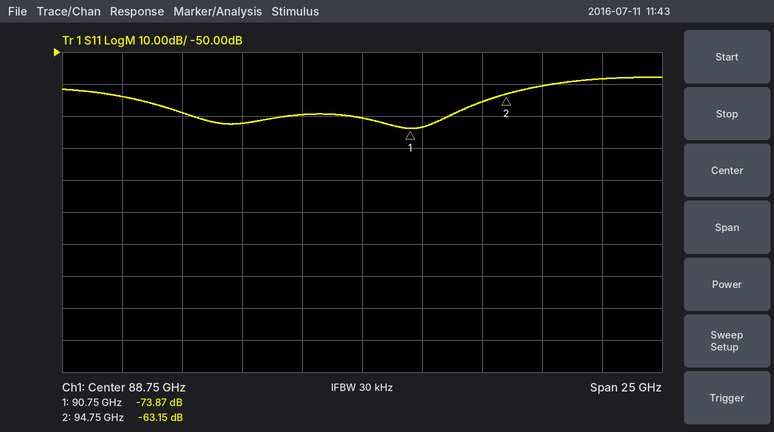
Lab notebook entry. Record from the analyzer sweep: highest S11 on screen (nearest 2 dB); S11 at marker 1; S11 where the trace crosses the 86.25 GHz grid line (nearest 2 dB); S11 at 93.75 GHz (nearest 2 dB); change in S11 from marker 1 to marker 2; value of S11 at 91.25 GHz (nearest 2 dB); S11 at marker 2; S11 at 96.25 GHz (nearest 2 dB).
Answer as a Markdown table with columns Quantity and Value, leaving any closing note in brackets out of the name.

| Quantity | Value |
|---|---|
| highest S11 on screen | -58 dB |
| S11 at marker 1 | -73.87 dB |
| S11 where the trace crosses the 86.25 GHz grid line | -70 dB |
| S11 at 93.75 GHz | -66 dB |
| change in S11 from marker 1 to marker 2 | 10.72 dB |
| value of S11 at 91.25 GHz | -74 dB |
| S11 at marker 2 | -63.15 dB |
| S11 at 96.25 GHz | -60 dB |
